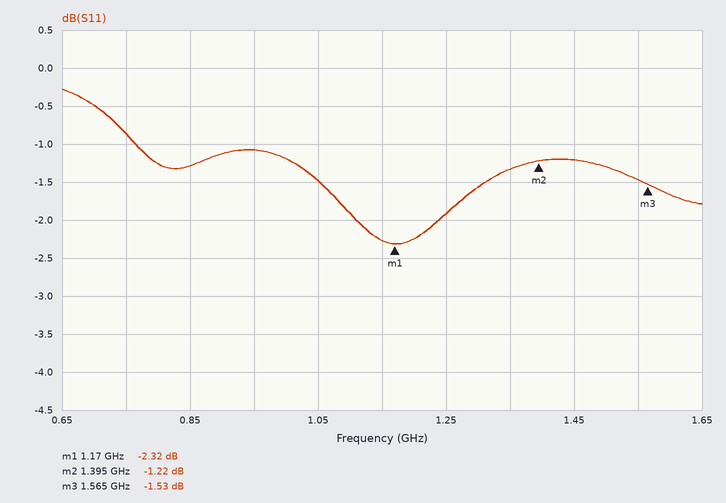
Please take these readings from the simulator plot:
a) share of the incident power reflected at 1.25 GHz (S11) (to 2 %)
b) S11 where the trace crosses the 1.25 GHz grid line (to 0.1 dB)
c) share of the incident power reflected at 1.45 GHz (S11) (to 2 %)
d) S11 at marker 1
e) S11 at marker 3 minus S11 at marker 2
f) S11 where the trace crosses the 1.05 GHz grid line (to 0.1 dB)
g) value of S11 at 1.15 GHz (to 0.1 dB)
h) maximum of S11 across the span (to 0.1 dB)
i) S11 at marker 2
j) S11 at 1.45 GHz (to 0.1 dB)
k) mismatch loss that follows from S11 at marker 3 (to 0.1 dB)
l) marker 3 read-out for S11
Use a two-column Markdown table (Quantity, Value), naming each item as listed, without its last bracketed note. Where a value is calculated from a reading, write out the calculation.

| Quantity | Value |
|---|---|
| share of the incident power reflected at 1.25 GHz (S11) | 10^(-1.9/10) ≈ 64.6 %, so 64 % to the nearest 2 % |
| S11 where the trace crosses the 1.25 GHz grid line | -1.9 dB |
| share of the incident power reflected at 1.45 GHz (S11) | 10^(-1.2/10) ≈ 76 % |
| S11 at marker 1 | -2.32 dB |
| S11 at marker 3 minus S11 at marker 2 | -1.53 − (-1.22) = -0.31 dB |
| S11 where the trace crosses the 1.05 GHz grid line | -1.5 dB |
| value of S11 at 1.15 GHz | -2.3 dB |
| maximum of S11 across the span | -0.3 dB |
| S11 at marker 2 | -1.22 dB |
| S11 at 1.45 GHz | -1.2 dB |
| mismatch loss that follows from S11 at marker 3 | −10 log10(1 − 10^(-1.53/10)) ≈ 5.3 dB |
| marker 3 read-out for S11 | -1.53 dB |
